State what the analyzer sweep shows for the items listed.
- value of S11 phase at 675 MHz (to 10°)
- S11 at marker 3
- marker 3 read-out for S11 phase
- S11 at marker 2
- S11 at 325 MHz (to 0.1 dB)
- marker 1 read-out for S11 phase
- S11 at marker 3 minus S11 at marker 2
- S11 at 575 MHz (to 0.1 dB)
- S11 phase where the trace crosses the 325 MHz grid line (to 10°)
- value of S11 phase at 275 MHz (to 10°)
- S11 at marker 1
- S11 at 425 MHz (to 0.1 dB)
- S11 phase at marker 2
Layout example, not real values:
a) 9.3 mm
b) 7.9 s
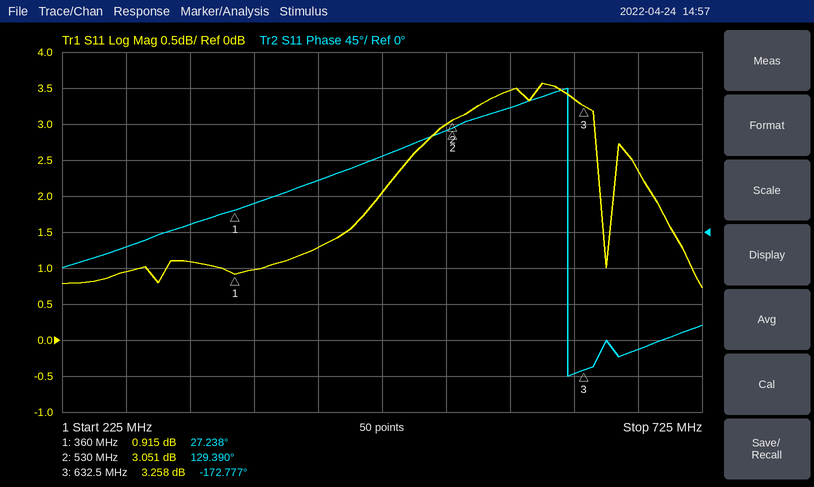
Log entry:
a) -150°
b) 3.258 dB
c) -172.777°
d) 3.051 dB
e) 1.1 dB
f) 27.238°
g) 0.207 dB
h) 3.5 dB
i) 10°
j) -20°
k) 0.915 dB
l) 1.3 dB
m) 129.390°
